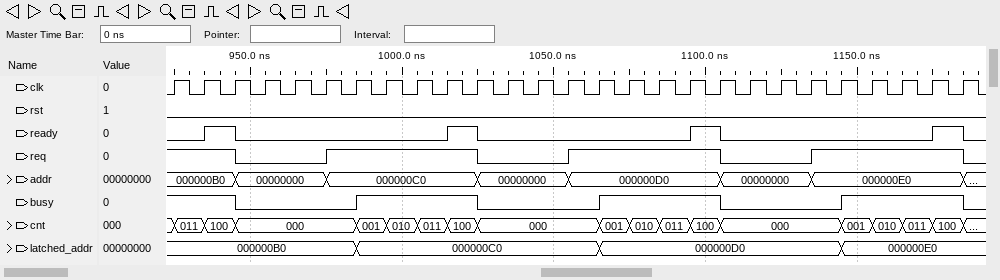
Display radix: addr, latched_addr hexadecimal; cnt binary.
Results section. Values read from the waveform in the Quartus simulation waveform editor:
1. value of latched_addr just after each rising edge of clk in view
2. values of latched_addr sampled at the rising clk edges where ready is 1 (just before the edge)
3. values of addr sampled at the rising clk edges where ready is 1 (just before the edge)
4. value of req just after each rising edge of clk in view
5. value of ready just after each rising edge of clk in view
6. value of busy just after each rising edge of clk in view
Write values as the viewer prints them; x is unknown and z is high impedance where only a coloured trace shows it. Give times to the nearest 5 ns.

000000B0, 000000B0, 000000B0, 000000B0, 000000B0, 000000B0, 000000C0, 000000C0, 000000C0, 000000C0, 000000C0, 000000C0, 000000C0, 000000C0, 000000D0, 000000D0, 000000D0, 000000D0, 000000D0, 000000D0, 000000D0, 000000D0, 000000E0, 000000E0, 000000E0, 000000E0, 000000E0
000000B0, 000000C0, 000000D0, 000000E0
000000B0, 000000C0, 000000D0, 000000E0
1 1 0 0 0 1 1 1 1 1 0 0 0 1 1 1 1 1 0 0 0 1 1 1 1 1 0
0 1 0 0 0 0 0 0 0 1 0 0 0 0 0 0 0 1 0 0 0 0 0 0 0 1 0
1 1 0 0 0 0 1 1 1 1 0 0 0 0 1 1 1 1 0 0 0 0 1 1 1 1 0
